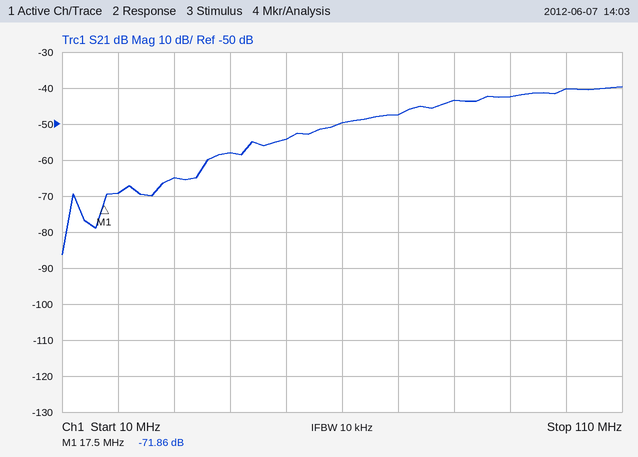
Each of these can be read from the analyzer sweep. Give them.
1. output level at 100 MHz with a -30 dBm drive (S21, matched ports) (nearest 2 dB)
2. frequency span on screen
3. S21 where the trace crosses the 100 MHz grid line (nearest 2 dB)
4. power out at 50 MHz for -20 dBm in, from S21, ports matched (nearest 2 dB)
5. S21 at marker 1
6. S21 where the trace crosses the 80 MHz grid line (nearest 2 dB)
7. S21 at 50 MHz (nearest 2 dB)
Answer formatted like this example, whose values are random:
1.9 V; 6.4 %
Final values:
-70 dBm; 100 MHz; -40 dB; -74 dBm; -71.86 dB; -44 dB; -54 dB
